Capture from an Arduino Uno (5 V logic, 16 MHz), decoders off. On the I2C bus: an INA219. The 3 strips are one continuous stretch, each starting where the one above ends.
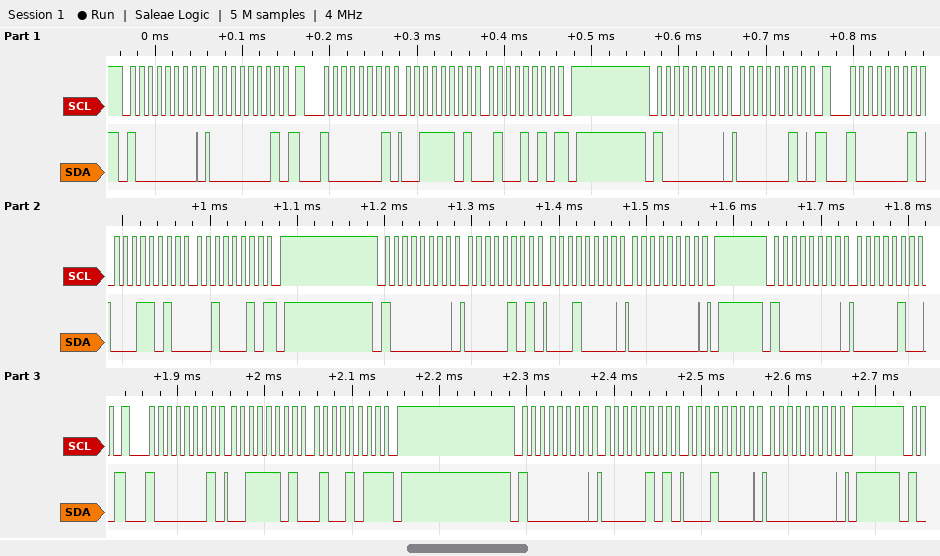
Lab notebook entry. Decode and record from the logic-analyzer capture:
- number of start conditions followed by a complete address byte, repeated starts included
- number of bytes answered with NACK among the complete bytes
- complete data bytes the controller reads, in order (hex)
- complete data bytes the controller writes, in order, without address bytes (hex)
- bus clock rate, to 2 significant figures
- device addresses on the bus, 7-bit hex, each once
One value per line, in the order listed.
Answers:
8
3
3D 4A 1A 22 3D 4B
01 02 05 10 00 04 05 10 00
100 kHz
0x40
